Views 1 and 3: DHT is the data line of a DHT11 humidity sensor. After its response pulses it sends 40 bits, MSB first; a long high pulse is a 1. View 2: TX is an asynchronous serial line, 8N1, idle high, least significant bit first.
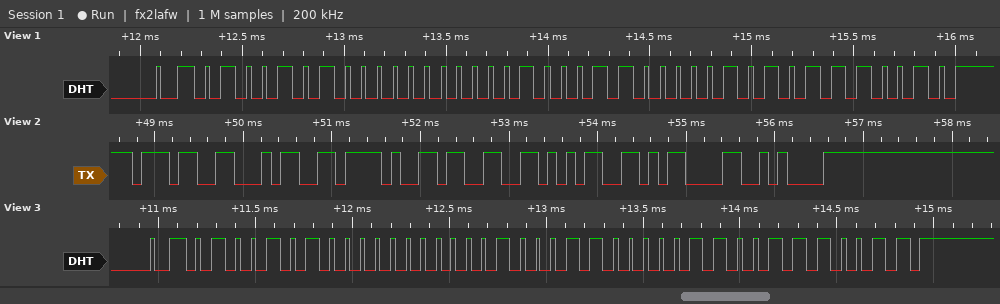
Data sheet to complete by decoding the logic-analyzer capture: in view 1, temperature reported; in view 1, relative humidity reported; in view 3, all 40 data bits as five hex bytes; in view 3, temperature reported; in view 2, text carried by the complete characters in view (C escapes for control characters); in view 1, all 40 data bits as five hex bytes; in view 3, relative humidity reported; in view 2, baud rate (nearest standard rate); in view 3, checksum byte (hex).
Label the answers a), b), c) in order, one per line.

a) 35.5 °C
b) 74 %
c) 4A 00 23 06 73
d) 35.6 °C
e) "74/35\r\n"
f) 4A 00 23 05 72
g) 74 %
h) 9600 baud
i) 0x73
